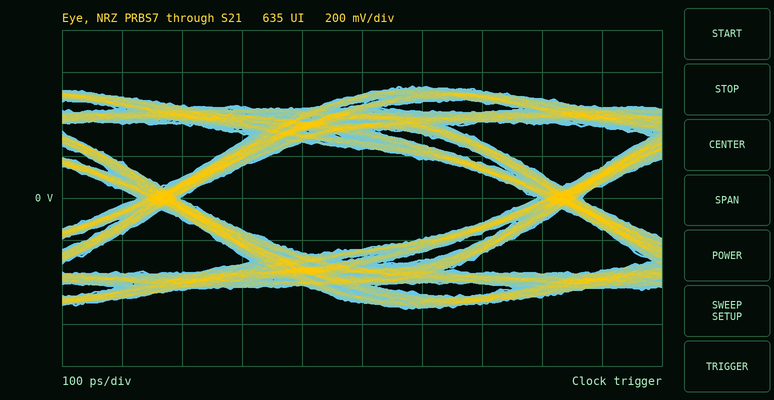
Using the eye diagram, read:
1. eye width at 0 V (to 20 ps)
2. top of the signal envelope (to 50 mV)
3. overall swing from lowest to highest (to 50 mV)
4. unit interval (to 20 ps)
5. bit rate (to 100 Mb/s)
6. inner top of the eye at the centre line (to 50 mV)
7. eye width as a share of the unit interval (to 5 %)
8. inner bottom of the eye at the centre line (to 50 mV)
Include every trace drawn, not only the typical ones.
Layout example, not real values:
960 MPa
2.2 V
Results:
600 ps
550 mV
1.05 V
660 ps
1.5 Gb/s
250 mV
90 %
-250 mV
